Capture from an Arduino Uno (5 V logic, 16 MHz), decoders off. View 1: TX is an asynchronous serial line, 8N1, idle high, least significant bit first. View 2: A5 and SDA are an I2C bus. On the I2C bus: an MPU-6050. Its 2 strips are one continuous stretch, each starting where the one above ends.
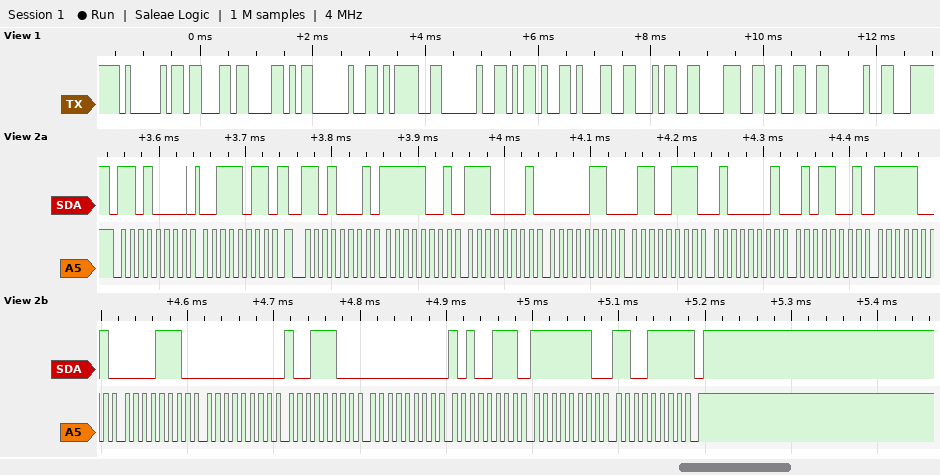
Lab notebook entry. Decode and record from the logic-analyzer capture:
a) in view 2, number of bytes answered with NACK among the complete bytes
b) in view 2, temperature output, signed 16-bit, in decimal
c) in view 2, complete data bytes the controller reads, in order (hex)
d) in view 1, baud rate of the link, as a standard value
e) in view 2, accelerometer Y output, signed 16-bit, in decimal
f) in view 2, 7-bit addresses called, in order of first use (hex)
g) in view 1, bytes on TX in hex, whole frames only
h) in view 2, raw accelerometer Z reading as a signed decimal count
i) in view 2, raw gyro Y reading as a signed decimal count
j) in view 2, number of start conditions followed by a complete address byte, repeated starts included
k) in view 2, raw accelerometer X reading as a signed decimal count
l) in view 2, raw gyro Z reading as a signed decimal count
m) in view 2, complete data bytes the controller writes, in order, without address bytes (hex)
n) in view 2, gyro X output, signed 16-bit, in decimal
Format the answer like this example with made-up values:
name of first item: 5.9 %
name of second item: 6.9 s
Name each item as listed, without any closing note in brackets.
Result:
in view 2, number of bytes answered with NACK among the complete bytes: 1
in view 2, temperature output, signed 16-bit, in decimal: -1778
in view 2, complete data bytes the controller reads, in order: F9 E1 06 67 41 59 F9 0E 00 9C 00 A7 FE CF
in view 1, baud rate of the link, as a standard value: 9600 baud
in view 2, accelerometer Y output, signed 16-bit, in decimal: 1639
in view 2, 7-bit addresses called, in order of first use: 0x68
in view 1, bytes on TX in hex, whole frames only: 41 63 58 20 3D 20 2D 31 34 38 32 20
in view 2, raw accelerometer Z reading as a signed decimal count: 16729
in view 2, raw gyro Y reading as a signed decimal count: 167
in view 2, number of start conditions followed by a complete address byte, repeated starts included: 2
in view 2, raw accelerometer X reading as a signed decimal count: -1567
in view 2, raw gyro Z reading as a signed decimal count: -305
in view 2, complete data bytes the controller writes, in order, without address bytes: 3B
in view 2, gyro X output, signed 16-bit, in decimal: 156
